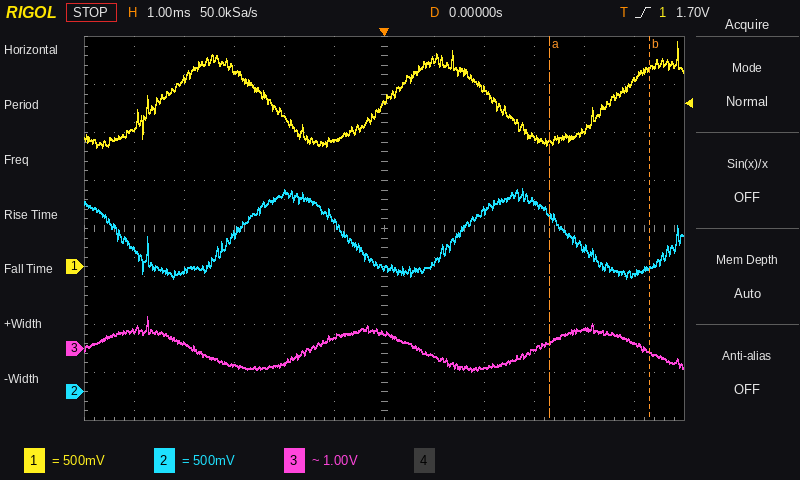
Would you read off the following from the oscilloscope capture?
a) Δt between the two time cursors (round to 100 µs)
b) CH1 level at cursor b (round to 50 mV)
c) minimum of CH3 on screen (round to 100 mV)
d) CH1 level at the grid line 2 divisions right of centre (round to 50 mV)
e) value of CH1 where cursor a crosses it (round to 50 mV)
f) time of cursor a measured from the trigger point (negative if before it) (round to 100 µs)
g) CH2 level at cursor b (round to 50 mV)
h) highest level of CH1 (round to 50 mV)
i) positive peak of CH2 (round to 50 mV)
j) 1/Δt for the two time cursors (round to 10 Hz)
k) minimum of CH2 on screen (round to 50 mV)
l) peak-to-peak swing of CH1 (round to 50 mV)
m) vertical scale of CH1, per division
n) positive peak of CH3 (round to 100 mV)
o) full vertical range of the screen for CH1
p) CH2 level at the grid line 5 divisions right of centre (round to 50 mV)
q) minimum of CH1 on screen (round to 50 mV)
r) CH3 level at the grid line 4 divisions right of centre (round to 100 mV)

2.0 ms
2.05 V
-500 mV
1.85 V
1.30 V
+3.3 ms
1.30 V
2.35 V
2.10 V
500 Hz
1.20 V
1.10 V
500 mV
700 mV
4 V
1.25 V
1.25 V
400 mV
